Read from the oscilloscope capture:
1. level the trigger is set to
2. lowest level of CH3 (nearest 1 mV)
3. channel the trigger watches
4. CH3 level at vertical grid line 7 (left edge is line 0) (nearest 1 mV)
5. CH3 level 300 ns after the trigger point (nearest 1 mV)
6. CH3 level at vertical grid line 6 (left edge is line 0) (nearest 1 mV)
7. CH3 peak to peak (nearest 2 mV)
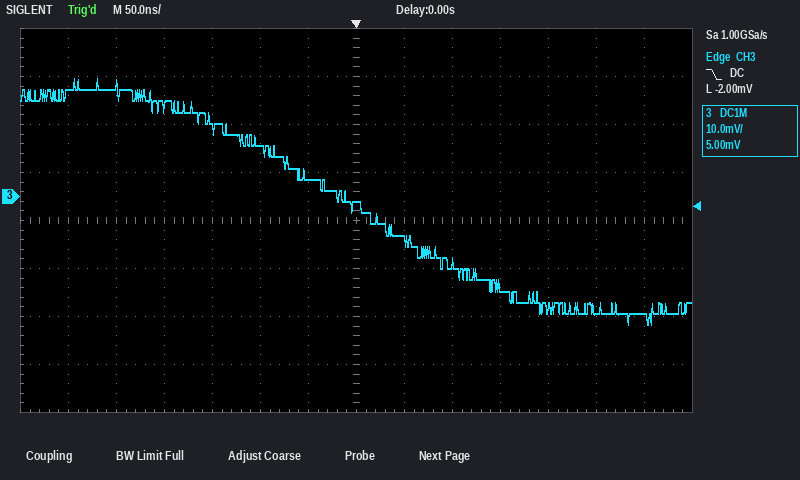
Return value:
-2.00 mV
-27 mV
CH3
-1 mV
-24 mV
4 mV
52 mV
